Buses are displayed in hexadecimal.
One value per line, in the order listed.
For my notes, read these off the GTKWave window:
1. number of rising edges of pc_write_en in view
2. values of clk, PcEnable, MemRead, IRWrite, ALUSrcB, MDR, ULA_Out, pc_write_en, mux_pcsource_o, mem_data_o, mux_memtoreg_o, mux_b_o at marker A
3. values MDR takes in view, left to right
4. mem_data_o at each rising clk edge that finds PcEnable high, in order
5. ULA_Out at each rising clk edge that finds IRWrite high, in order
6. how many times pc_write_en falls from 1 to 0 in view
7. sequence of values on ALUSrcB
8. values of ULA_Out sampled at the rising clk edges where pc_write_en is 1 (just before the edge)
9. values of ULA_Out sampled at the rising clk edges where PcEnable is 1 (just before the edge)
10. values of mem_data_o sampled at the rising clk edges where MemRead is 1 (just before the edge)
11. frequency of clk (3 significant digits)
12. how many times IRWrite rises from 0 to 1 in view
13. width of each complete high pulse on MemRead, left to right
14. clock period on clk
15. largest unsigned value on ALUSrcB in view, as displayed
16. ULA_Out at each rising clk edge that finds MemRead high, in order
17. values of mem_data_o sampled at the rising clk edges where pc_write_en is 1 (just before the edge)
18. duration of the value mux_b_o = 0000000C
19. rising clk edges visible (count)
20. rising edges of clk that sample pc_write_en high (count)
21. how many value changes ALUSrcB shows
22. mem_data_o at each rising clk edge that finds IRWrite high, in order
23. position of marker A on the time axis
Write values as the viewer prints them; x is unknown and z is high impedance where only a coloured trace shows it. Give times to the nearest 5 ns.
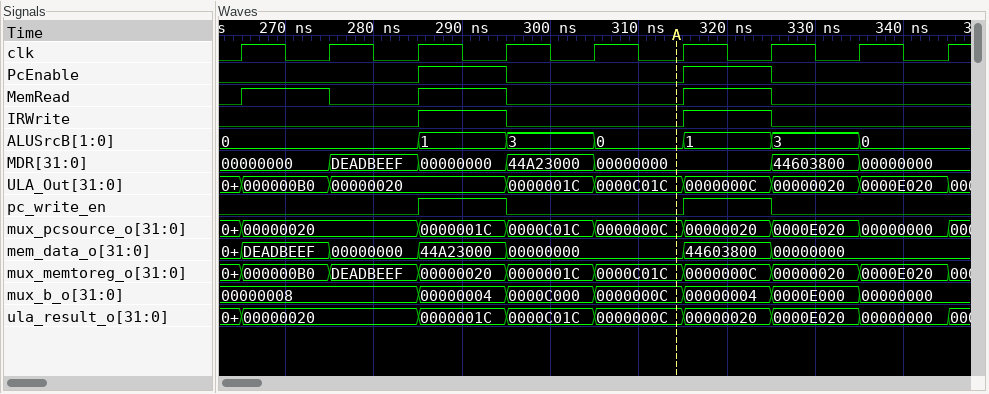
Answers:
2
clk=0, PcEnable=0, MemRead=0, IRWrite=0, ALUSrcB=0, MDR=00000000, ULA_Out=0000C01C, pc_write_en=0, mux_pcsource_o=0000000C, mem_data_o=00000000, mux_memtoreg_o=0000C01C, mux_b_o=0000000C
00000000, DEADBEEF, 00000000, 44A23000, 00000000, 44603800, 00000000
44A23000, 44603800
00000020, 0000000C
2
0, 1, 3, 0, 1, 3, 0
00000020, 0000000C
00000020, 0000000C
DEADBEEF, 44A23000, 44603800
100 MHz
2
10 ns, 10 ns, 10 ns
10 ns
3
000000B0, 00000020, 0000000C
44A23000, 44603800
10 ns
9
2
6
44A23000, 44603800
315 ns
